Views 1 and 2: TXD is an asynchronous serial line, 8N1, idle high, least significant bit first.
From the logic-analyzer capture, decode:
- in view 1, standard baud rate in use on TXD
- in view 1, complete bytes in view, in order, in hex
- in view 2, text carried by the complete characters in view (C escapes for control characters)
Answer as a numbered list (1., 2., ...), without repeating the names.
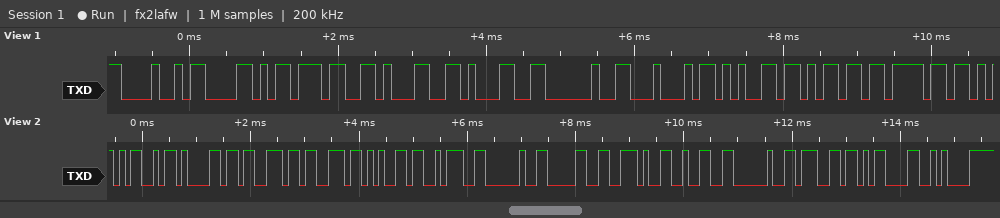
1. 9600 baud
2. 0x48 0x58 0x37 0x31 0x31 0x20 0x44 0x65 0x6D 0x6F
3. "Masse: 0.2 g\r\n"
